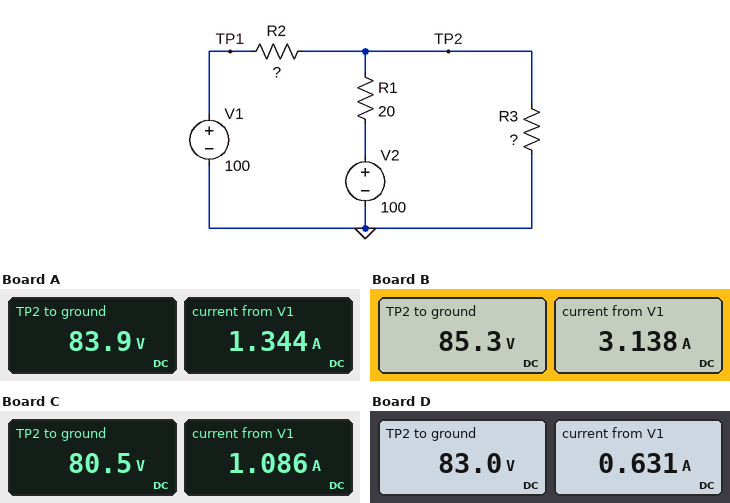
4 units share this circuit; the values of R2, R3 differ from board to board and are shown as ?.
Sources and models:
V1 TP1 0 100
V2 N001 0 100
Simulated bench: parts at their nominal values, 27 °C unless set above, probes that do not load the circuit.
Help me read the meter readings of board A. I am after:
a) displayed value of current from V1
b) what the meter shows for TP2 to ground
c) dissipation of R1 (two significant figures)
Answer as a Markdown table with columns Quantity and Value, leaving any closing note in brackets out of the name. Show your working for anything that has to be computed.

| Quantity | Value |
|---|---|
| displayed value of current from V1 | 1.344 A |
| what the meter shows for TP2 to ground | 83.9 V |
| dissipation of R1 | (100 V - 83.9 V)^2 / 20 Ω = 13 W |
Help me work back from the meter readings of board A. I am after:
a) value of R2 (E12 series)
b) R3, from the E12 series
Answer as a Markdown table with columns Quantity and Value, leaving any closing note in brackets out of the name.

| Quantity | Value |
|---|---|
| value of R2 | 12 Ω |
| R3, from the E12 series | 39 Ω |
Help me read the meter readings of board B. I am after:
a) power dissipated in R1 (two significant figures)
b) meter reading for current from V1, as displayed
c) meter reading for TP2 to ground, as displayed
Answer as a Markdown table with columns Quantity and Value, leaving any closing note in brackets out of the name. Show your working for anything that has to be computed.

| Quantity | Value |
|---|---|
| power dissipated in R1 | (100 V - 85.3 V)^2 / 20 Ω = 11 W |
| meter reading for current from V1, as displayed | 3.138 A |
| meter reading for TP2 to ground, as displayed | 85.3 V |
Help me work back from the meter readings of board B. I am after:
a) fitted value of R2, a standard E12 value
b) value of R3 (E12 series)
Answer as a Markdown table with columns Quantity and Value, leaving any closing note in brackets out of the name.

| Quantity | Value |
|---|---|
| fitted value of R2, a standard E12 value | 4.7 Ω |
| value of R3 | 22 Ω |
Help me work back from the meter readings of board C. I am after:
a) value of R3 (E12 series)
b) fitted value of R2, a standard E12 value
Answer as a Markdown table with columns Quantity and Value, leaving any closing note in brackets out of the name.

| Quantity | Value |
|---|---|
| value of R3 | 39 Ω |
| fitted value of R2, a standard E12 value | 18 Ω |
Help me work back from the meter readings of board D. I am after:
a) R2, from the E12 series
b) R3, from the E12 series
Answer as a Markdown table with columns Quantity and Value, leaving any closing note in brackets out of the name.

| Quantity | Value |
|---|---|
| R2, from the E12 series | 27 Ω |
| R3, from the E12 series | 56 Ω |
